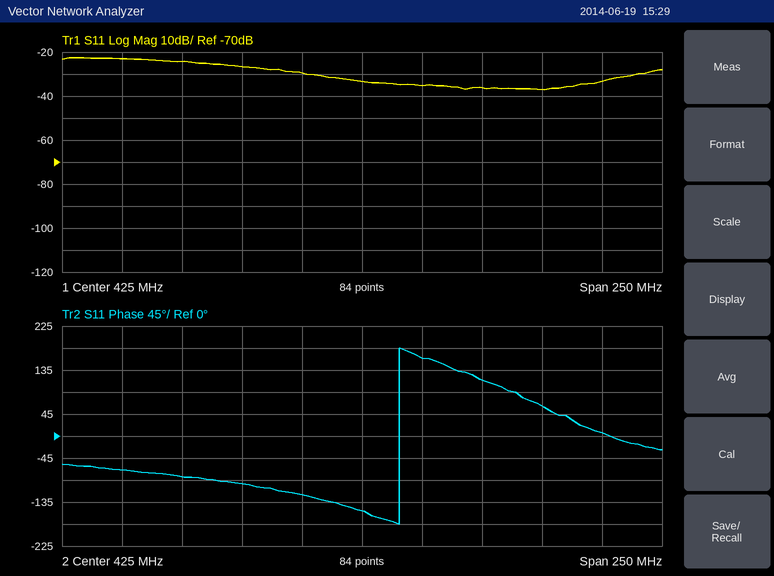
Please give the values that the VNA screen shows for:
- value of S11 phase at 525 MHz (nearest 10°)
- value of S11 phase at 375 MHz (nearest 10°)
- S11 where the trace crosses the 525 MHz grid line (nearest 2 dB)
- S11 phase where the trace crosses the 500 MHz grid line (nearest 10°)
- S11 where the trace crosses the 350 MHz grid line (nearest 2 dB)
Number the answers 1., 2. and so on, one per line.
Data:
1. 10°
2. -100°
3. -34 dB
4. 60°
5. -24 dB
